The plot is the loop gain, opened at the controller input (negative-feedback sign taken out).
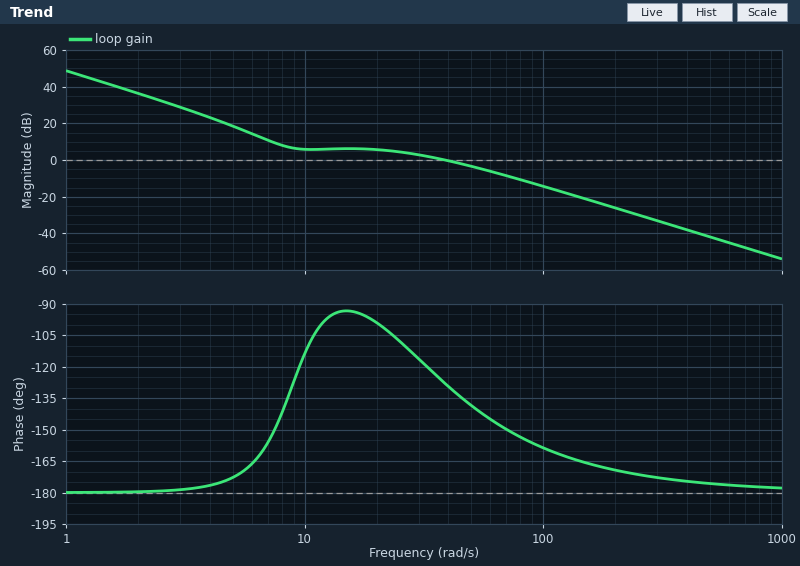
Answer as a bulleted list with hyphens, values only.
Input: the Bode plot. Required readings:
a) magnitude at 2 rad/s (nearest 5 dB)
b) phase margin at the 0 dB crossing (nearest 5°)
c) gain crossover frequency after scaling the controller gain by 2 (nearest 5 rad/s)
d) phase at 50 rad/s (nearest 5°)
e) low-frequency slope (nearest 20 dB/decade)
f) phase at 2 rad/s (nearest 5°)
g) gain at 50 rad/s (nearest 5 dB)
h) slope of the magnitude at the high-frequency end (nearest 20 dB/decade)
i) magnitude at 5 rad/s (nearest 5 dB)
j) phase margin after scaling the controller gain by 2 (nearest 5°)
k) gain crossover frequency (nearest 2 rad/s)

- 35 dB
- 50°
- 60 rad/s
- -140°
- -40 dB/decade
- -180°
- -5 dB
- -40 dB/decade
- 20 dB
- 35°
- 38 rad/s
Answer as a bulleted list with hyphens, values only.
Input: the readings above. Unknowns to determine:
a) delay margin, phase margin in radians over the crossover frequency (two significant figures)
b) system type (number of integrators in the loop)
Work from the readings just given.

- 0.023 s
- 2
